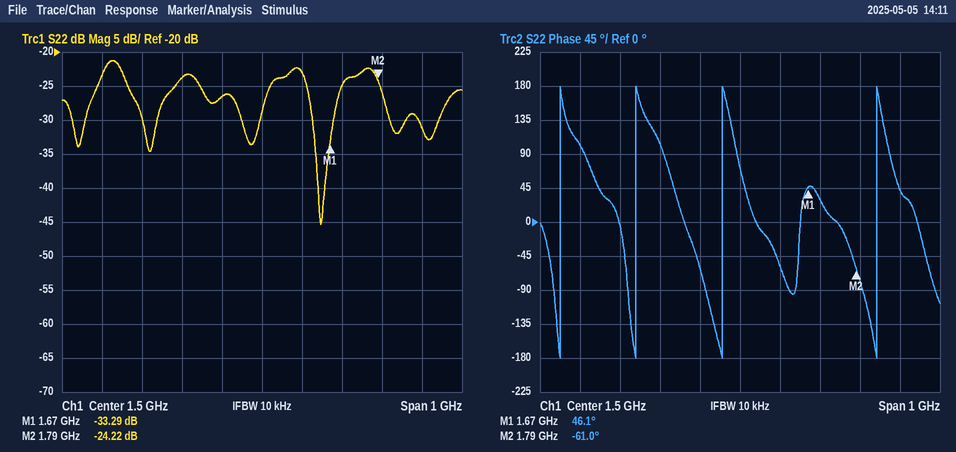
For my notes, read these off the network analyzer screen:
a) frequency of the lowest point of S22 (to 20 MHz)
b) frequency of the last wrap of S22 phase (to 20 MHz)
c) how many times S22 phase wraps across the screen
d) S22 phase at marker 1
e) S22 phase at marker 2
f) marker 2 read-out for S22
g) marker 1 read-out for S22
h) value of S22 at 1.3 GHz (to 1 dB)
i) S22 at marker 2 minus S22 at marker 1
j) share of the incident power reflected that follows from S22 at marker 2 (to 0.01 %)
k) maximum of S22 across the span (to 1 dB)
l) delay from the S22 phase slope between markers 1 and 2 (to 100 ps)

1.64 GHz
1.84 GHz
4
46.1°
-61.0°
-24.22 dB
-33.29 dB
-24 dB
9.07 dB
0.38 %
-21 dB
2.5 ns
